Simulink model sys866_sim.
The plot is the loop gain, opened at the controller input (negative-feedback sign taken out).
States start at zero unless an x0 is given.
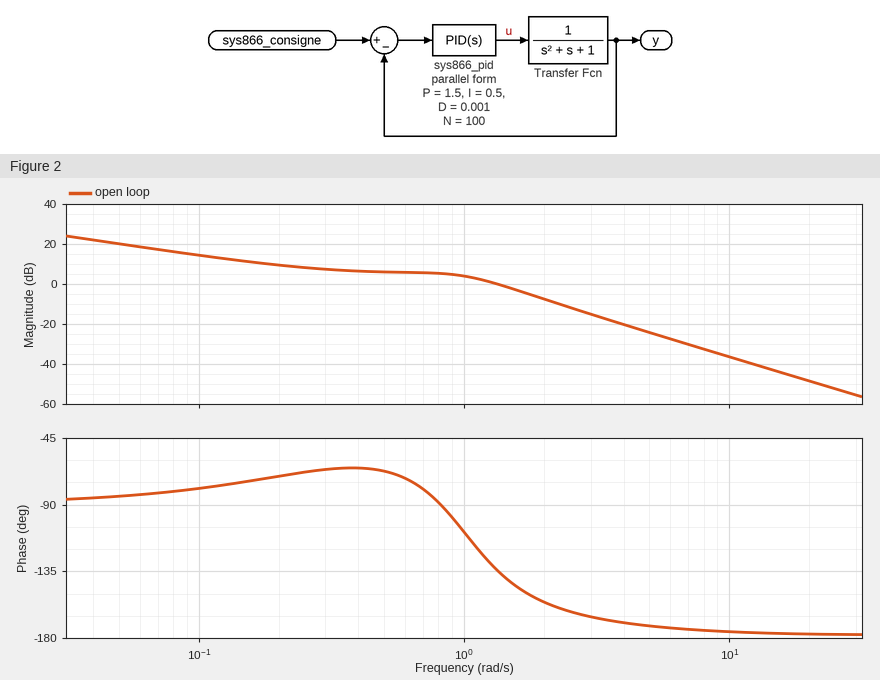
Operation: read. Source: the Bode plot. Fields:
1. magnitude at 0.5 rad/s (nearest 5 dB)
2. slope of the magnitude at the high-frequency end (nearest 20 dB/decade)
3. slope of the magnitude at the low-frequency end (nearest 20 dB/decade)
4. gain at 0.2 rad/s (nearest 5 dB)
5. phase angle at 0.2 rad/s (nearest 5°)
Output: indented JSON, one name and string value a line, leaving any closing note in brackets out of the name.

{
  "magnitude at 0.5 rad/s": "5 dB",
  "slope of the magnitude at the high-frequency end": "-40 dB/decade",
  "slope of the magnitude at the low-frequency end": "-20 dB/decade",
  "gain at 0.2 rad/s": "10 dB",
  "phase angle at 0.2 rad/s": "-70°"
}
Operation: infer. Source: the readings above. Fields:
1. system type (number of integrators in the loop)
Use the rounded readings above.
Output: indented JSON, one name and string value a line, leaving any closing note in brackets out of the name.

{
  "system type": "1"
}
